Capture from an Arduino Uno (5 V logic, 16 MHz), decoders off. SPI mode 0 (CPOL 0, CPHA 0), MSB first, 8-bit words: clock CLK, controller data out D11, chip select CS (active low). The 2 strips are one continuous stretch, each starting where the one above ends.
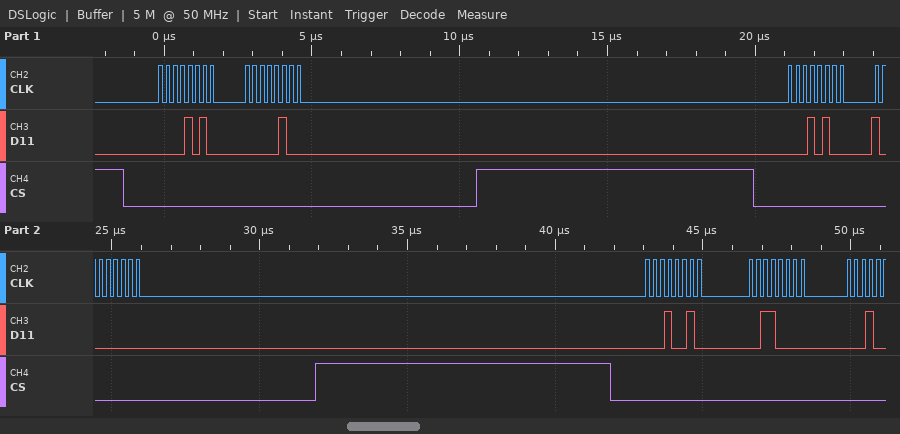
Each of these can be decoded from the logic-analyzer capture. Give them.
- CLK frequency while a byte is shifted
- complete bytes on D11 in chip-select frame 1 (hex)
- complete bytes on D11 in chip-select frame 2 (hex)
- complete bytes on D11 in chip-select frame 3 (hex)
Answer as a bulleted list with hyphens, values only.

- 4 MHz
- 0A 04
- 14 80
- 12 30
